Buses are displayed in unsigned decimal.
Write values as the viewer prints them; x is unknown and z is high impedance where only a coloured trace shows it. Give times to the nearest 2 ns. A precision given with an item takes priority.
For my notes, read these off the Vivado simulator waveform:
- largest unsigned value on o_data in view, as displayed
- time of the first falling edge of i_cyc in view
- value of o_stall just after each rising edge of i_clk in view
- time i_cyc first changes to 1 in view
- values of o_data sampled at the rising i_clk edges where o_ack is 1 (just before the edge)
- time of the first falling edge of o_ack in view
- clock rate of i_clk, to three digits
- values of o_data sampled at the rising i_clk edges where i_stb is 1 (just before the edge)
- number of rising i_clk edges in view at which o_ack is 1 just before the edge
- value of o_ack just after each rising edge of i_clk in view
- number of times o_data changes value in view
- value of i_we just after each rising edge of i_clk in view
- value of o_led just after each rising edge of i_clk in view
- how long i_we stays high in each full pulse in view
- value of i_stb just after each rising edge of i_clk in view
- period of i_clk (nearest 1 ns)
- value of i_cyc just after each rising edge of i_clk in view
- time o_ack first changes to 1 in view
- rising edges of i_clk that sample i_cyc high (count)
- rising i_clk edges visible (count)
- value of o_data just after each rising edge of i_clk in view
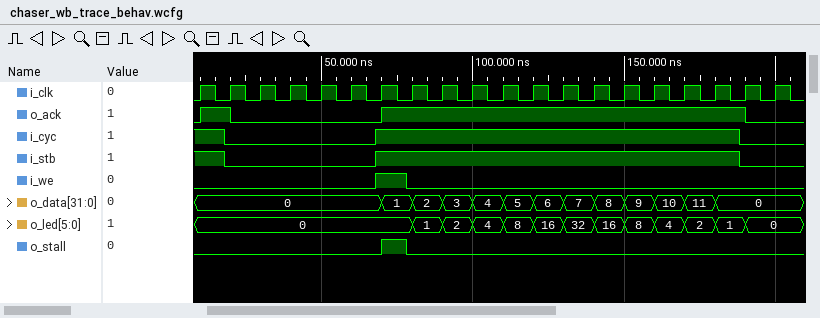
11
18 ns
0 0 0 0 0 0 1 0 0 0 0 0 0 0 0 0 0 0 0 0
68 ns
0, 1, 2, 3, 4, 5, 6, 7, 8, 9, 10, 11, 0
20 ns
100 MHz
0, 0, 1, 2, 3, 4, 5, 6, 7, 8, 9, 10, 11
13
1 0 0 0 0 0 1 1 1 1 1 1 1 1 1 1 1 1 0 0
12
0 0 0 0 0 0 1 0 0 0 0 0 0 0 0 0 0 0 0 0
0, 0, 0, 0, 0, 0, 0, 1, 2, 4, 8, 16, 32, 16, 8, 4, 2, 1, 0, 0
10 ns
1 0 0 0 0 0 1 1 1 1 1 1 1 1 1 1 1 1 0 0
10 ns
1 0 0 0 0 0 1 1 1 1 1 1 1 1 1 1 1 1 0 0
10 ns
13
20
0, 0, 0, 0, 0, 0, 1, 2, 3, 4, 5, 6, 7, 8, 9, 10, 11, 0, 0, 0
